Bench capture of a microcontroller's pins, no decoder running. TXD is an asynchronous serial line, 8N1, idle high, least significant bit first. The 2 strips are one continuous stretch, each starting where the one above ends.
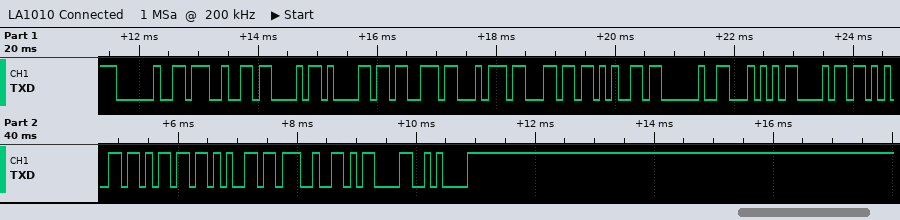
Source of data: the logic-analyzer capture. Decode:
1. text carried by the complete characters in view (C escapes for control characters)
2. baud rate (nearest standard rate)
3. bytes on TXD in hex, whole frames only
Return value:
" 'Castle Theme'\r\n"
9600 baud
20 27 43 61 73 74 6C 65 20 54 68 65 6D 65 27 0D 0A
